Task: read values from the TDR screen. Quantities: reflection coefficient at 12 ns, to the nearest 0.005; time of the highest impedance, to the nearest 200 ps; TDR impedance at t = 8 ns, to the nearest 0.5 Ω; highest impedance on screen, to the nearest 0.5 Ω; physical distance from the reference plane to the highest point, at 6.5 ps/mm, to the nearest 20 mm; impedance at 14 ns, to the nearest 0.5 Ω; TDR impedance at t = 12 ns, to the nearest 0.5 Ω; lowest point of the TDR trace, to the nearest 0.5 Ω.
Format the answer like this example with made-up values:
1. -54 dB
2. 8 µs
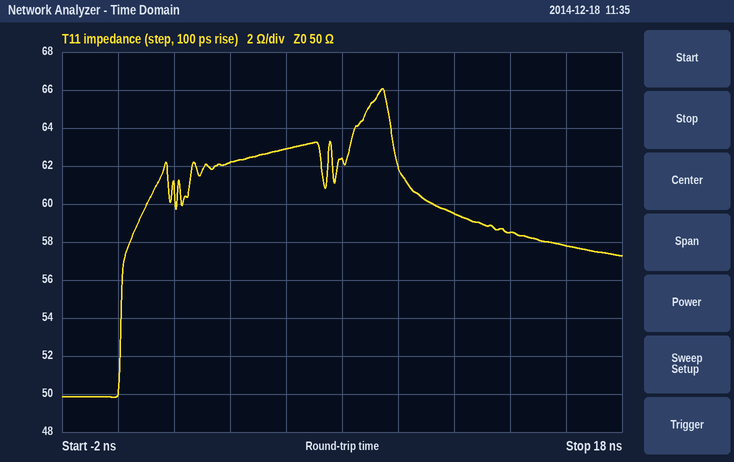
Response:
1. +0.085
2. 9.4 ns
3. 62.5 Ω
4. 66.0 Ω
5. 720 mm
6. 58.5 Ω
7. 59.5 Ω
8. 50.0 Ω
